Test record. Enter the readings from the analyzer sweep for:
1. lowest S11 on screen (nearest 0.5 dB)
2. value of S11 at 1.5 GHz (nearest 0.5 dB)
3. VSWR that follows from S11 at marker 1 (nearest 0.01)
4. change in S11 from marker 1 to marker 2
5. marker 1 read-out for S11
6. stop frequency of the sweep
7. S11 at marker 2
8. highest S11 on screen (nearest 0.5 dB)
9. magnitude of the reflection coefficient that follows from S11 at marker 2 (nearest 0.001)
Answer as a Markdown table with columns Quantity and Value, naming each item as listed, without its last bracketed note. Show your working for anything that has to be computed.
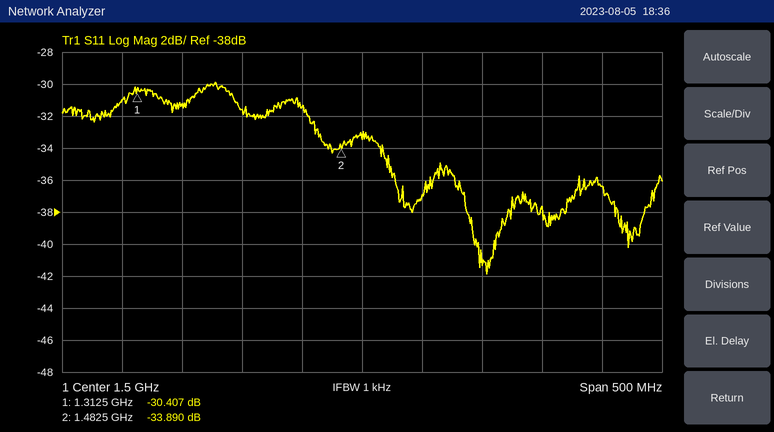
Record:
| Quantity | Value |
|---|---|
| lowest S11 on screen | -42.0 dB |
| value of S11 at 1.5 GHz | -33.5 dB |
| VSWR that follows from S11 at marker 1 | (1 + 0.0302)/(1 − 0.0302) ≈ 1.06 |
| change in S11 from marker 1 to marker 2 | -33.89 − (-30.407) = -3.483 dB |
| marker 1 read-out for S11 | -30.407 dB |
| stop frequency of the sweep | 1.75 GHz |
| S11 at marker 2 | -33.890 dB |
| highest S11 on screen | -30.0 dB |
| magnitude of the reflection coefficient that follows from S11 at marker 2 | 10^(-33.89/20) ≈ 0.020 |
